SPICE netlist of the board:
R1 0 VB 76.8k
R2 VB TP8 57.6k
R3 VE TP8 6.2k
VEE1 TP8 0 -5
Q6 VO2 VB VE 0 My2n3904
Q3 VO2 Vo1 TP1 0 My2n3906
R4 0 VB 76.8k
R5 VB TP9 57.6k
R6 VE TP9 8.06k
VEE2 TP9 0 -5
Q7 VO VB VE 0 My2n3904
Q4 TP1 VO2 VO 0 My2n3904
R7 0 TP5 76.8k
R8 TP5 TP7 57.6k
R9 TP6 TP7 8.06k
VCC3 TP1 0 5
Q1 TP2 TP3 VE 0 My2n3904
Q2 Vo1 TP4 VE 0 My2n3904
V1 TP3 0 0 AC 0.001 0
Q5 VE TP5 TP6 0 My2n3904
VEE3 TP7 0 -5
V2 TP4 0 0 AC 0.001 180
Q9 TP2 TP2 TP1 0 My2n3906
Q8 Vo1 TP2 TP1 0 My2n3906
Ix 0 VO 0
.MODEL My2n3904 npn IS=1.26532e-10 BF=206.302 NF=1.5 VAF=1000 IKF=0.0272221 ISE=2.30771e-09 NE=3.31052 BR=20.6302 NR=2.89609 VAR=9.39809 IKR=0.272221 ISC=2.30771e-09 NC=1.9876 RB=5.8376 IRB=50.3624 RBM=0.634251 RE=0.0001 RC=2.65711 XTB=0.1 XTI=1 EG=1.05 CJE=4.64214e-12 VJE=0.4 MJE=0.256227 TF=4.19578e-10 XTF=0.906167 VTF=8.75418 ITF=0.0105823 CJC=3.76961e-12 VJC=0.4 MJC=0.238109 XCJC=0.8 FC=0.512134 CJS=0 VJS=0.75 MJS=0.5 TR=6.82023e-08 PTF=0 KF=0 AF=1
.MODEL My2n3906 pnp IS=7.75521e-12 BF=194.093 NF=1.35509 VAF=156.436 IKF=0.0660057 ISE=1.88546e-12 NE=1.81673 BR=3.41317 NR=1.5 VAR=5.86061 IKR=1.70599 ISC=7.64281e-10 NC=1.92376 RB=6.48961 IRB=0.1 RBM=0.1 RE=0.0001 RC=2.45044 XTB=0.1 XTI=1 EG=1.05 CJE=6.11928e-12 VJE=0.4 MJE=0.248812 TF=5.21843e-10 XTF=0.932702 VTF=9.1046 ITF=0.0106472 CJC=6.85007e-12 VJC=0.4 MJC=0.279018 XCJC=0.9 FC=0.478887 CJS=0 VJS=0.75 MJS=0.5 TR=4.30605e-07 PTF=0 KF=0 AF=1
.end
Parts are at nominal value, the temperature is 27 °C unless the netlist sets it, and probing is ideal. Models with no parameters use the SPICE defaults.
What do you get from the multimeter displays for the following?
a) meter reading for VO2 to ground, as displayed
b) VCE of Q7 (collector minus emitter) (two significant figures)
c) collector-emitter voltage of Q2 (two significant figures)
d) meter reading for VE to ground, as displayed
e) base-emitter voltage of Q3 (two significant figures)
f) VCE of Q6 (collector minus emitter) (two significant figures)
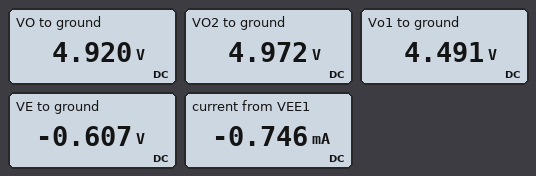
4.972 V
5.5 V
5.1 V
-0.607 V
-510 mV
5.6 V
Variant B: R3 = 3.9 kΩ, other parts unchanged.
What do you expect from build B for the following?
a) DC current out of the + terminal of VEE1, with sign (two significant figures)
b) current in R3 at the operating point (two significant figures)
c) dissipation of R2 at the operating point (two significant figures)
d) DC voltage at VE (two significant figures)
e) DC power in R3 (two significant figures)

-1.2 mA
1.1 mA
80 µW
-620 mV
4.9 mW
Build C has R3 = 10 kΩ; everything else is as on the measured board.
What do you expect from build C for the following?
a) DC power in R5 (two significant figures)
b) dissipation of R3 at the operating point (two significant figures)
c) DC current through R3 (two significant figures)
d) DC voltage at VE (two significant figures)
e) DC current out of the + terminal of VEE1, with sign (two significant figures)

80 µW
1.9 mW
440 µA
-600 mV
-480 µA
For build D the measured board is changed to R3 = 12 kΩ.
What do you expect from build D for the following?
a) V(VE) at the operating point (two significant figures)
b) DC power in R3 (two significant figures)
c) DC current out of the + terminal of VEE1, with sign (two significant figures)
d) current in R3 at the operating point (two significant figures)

-600 mV
1.6 mW
-400 µA
370 µA
